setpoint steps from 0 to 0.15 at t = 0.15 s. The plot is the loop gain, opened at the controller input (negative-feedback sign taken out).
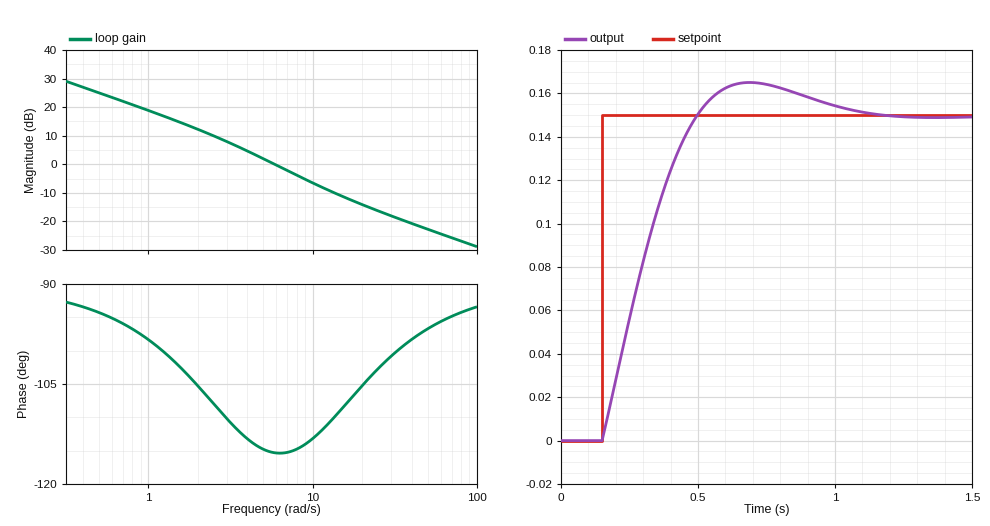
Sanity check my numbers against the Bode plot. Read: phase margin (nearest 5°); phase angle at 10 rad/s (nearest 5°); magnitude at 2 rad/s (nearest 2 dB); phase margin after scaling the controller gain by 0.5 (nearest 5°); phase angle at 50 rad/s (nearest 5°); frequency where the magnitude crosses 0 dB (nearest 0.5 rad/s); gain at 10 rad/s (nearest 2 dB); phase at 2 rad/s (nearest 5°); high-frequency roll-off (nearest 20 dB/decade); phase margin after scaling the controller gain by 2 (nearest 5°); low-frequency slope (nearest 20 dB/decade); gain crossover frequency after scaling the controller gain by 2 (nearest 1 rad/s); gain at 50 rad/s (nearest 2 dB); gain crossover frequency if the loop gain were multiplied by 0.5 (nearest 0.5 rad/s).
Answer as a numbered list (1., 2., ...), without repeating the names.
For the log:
1. 65°
2. -115°
3. 12 dB
4. 70°
5. -95°
6. 6.0 rad/s
7. -6 dB
8. -105°
9. -20 dB/decade
10. 65°
11. -20 dB/decade
12. 10 rad/s
13. -22 dB
14. 3.5 rad/s
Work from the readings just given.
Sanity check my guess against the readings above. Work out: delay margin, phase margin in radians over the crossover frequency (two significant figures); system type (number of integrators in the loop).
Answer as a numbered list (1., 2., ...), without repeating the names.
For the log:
1. 0.19 s
2. 1
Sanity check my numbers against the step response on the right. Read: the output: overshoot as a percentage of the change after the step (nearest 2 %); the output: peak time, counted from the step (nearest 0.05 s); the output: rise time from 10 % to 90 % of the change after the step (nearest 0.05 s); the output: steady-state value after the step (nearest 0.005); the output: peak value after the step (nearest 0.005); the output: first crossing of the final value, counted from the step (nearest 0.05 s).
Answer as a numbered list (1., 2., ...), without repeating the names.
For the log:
1. 10 %
2. 0.55 s
3. 0.25 s
4. 0.150
5. 0.165
6. 0.35 s
